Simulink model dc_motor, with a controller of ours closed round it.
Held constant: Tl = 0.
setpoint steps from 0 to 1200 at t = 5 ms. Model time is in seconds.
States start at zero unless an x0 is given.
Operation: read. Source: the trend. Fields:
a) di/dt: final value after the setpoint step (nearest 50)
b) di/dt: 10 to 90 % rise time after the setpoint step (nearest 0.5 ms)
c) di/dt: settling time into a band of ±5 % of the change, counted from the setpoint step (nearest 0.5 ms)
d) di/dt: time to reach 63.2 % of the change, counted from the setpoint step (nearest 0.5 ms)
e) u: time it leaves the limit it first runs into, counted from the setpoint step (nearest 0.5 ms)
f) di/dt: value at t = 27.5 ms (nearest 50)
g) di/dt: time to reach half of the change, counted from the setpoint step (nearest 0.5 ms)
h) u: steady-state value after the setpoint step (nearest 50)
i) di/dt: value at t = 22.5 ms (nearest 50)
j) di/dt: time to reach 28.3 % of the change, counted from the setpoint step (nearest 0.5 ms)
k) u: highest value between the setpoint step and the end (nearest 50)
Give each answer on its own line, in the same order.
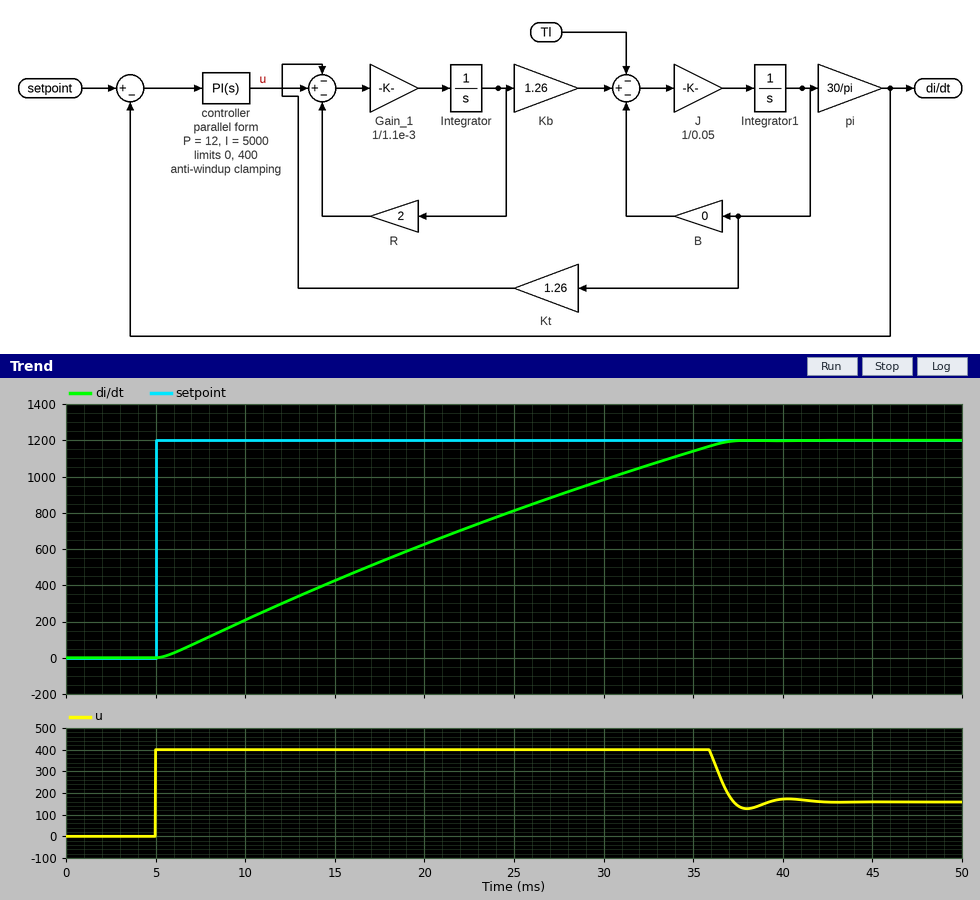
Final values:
1200
25.0 ms
30.0 ms
18.5 ms
31.0 ms
900
14.5 ms
150
700
8.0 ms
400
